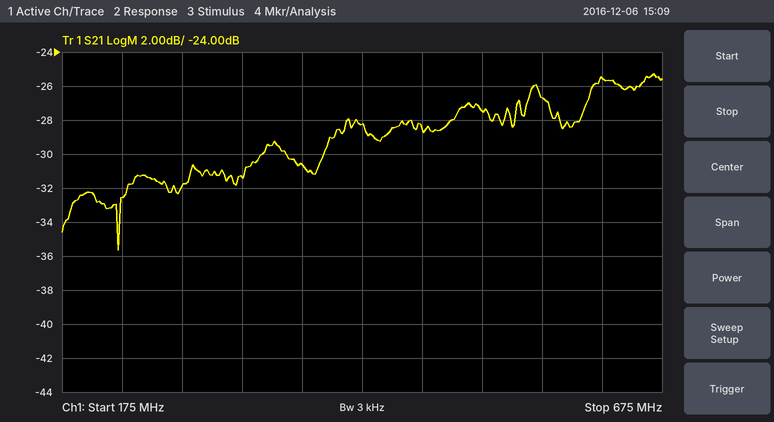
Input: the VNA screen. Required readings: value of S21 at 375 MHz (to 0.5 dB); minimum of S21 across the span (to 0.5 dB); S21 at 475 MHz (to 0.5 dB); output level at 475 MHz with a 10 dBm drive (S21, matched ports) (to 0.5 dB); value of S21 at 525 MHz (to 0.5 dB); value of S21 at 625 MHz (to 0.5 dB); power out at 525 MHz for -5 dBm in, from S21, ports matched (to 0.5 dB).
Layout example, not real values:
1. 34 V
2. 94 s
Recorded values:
1. -30.5 dB
2. -35.5 dB
3. -28.5 dB
4. -18.5 dBm
5. -27.5 dB
6. -25.5 dB
7. -32.5 dBm
